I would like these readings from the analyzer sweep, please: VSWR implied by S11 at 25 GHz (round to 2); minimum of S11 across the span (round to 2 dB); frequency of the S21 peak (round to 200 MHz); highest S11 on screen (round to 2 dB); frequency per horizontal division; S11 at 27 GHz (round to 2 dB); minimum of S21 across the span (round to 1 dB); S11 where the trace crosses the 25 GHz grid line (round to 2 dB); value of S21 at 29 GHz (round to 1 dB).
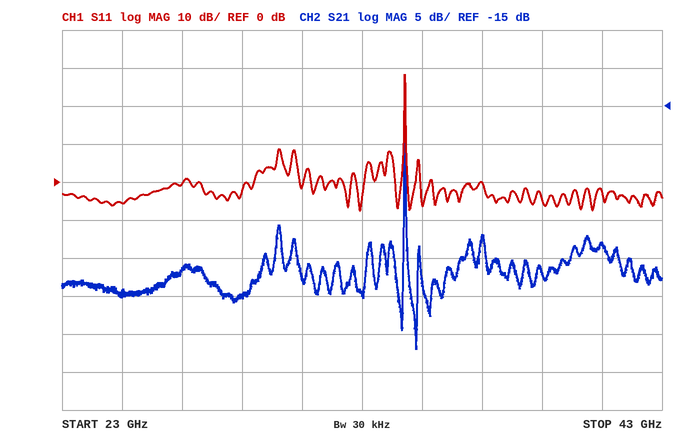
4
-8 dB
34.4 GHz
28 dB
2 GHz
0 dB
-47 dB
-6 dB
-40 dB
